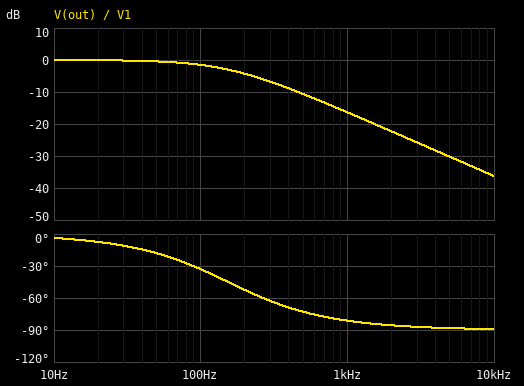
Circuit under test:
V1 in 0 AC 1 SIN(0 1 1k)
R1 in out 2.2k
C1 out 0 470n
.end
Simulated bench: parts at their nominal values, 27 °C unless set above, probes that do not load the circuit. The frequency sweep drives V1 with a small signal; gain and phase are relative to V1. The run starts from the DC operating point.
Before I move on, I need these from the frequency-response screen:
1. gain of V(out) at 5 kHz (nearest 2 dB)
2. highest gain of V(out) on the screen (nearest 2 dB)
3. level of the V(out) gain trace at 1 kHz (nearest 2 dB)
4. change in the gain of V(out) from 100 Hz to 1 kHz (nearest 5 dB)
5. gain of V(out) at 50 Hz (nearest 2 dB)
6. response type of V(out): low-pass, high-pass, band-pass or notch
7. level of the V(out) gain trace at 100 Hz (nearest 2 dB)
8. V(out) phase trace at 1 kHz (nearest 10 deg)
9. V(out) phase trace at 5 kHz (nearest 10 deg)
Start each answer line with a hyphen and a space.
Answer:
- -30 dB
- 0 dB
- -16 dB
- -15 dB
- 0 dB
- low-pass
- -2 dB
- -80 deg
- -90 deg
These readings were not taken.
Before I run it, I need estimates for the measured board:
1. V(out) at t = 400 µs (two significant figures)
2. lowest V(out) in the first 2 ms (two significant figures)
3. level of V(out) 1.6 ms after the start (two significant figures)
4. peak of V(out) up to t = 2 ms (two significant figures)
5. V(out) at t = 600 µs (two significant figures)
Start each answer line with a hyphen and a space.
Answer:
- 240 mV
- -130 mV
- 140 mV
- 250 mV
- 190 mV
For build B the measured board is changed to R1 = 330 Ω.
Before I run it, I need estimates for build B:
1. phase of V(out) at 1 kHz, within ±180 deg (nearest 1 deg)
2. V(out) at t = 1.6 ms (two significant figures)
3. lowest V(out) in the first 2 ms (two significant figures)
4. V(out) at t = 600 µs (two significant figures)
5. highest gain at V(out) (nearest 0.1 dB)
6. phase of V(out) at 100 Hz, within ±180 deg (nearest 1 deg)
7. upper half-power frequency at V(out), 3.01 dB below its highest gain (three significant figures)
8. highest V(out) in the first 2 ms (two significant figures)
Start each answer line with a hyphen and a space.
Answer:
- -44 deg
- 100 mV
- -720 mV
- 110 mV
- 0 dB
- -6 deg
- 1.03 kHz
- 760 mV
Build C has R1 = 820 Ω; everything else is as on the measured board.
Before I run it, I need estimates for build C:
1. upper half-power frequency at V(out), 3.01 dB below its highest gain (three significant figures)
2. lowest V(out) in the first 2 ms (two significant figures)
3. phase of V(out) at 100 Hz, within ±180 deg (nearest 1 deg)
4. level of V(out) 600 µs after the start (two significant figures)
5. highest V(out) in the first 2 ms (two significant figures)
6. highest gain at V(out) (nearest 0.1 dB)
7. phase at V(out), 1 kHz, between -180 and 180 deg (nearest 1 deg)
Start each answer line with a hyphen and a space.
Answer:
- 413 Hz
- -380 mV
- -14 deg
- 270 mV
- 500 mV
- 0 dB
- -68 deg
